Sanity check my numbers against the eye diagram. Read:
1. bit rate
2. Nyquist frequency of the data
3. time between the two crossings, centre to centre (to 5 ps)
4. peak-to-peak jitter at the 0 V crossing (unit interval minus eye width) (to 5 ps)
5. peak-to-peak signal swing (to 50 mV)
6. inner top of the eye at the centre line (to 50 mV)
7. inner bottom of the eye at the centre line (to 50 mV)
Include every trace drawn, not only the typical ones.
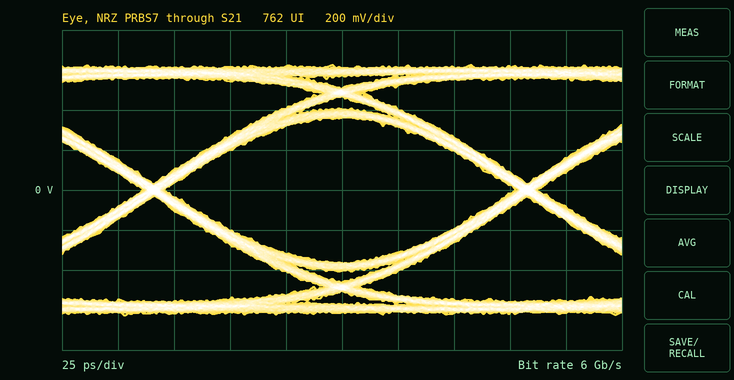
6 Gb/s
3 GHz
165 ps
10 ps
1.25 V
350 mV
-350 mV
